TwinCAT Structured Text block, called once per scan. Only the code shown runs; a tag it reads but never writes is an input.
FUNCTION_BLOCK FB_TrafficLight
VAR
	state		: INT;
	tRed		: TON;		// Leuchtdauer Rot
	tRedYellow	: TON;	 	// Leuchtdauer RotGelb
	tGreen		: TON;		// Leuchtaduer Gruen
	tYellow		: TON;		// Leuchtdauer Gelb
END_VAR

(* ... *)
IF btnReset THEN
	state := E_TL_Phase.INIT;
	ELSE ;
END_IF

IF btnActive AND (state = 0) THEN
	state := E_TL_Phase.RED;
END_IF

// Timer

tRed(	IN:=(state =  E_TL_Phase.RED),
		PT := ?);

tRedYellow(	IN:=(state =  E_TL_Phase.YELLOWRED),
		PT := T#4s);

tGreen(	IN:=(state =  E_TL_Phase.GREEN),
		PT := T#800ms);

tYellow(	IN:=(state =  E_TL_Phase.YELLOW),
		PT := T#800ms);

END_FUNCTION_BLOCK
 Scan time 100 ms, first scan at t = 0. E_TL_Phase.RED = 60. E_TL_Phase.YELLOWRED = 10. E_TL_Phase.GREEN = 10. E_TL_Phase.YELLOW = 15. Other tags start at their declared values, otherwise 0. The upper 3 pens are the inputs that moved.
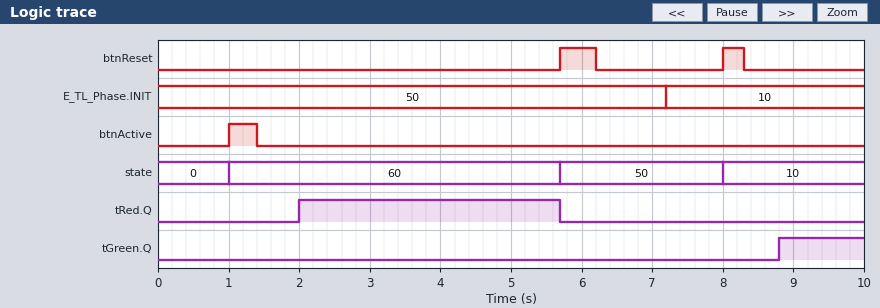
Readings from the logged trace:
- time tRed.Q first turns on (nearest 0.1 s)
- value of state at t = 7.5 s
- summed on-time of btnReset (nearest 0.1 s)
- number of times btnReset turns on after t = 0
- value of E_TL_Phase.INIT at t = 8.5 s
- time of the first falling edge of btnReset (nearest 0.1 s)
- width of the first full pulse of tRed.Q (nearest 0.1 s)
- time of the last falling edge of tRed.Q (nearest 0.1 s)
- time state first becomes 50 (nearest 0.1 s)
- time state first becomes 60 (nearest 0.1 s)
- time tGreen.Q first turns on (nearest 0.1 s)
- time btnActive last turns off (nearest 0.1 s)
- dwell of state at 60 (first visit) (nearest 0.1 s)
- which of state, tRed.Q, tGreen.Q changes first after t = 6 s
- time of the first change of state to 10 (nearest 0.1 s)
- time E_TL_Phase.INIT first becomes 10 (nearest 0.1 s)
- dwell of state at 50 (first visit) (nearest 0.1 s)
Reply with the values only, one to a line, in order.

2.0 s
50
0.8 s
2
10
6.2 s
3.7 s
5.7 s
5.7 s
1.0 s
8.8 s
1.4 s
4.7 s
state
8.0 s
7.2 s
2.3 s
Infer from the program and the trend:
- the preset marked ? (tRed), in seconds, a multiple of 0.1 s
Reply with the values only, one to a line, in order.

1.0 s
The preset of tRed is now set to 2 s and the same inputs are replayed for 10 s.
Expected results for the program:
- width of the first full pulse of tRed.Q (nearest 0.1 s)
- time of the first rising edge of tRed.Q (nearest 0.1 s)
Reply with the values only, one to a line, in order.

2.7 s
3.0 s
